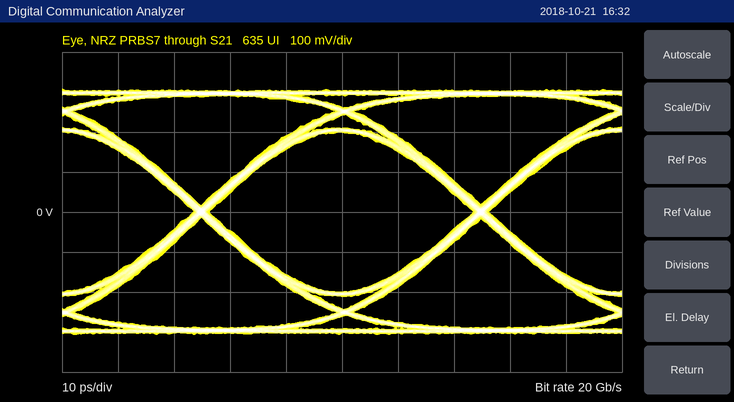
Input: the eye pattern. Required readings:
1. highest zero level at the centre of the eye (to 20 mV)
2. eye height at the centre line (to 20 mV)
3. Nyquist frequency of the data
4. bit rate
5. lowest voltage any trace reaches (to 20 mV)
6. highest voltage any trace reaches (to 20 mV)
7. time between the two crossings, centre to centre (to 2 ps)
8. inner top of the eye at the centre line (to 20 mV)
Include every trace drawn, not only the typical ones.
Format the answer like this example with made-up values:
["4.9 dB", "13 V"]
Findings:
["-200 mV", "400 mV", "10 GHz", "20 Gb/s", "-300 mV", "300 mV", "50 ps", "200 mV"]
